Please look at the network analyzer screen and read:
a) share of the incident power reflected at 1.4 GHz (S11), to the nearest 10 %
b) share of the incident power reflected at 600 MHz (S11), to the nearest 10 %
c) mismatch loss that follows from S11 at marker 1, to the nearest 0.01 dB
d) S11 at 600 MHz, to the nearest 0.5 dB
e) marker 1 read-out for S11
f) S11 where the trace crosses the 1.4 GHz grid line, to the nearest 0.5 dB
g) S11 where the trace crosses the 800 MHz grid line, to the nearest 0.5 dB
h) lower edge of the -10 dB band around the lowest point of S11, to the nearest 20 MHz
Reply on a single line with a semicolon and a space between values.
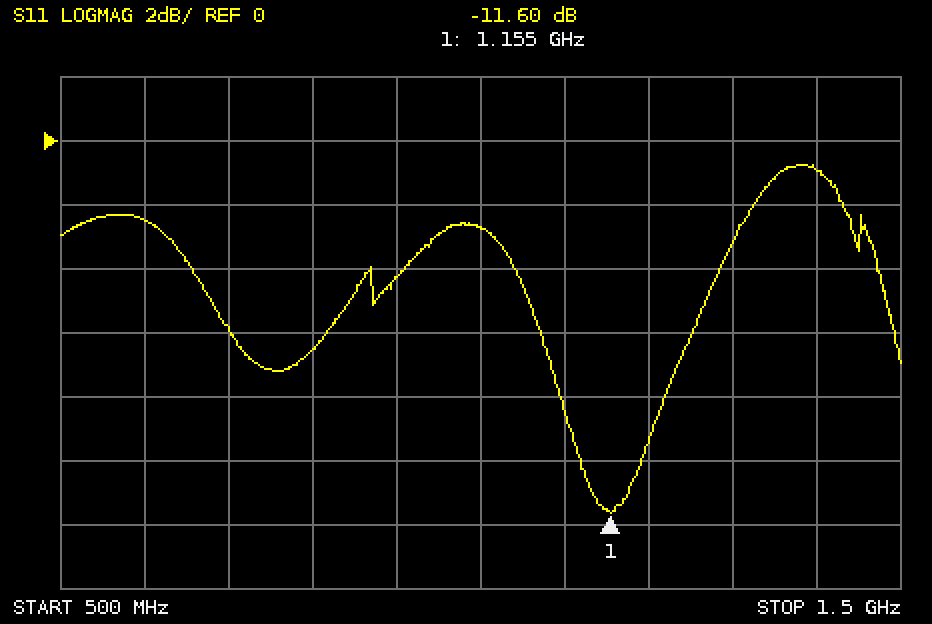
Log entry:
80 %; 60 %; 0.31 dB; -2.5 dB; -11.60 dB; -1.0 dB; -6.5 dB; 1.12 GHz
